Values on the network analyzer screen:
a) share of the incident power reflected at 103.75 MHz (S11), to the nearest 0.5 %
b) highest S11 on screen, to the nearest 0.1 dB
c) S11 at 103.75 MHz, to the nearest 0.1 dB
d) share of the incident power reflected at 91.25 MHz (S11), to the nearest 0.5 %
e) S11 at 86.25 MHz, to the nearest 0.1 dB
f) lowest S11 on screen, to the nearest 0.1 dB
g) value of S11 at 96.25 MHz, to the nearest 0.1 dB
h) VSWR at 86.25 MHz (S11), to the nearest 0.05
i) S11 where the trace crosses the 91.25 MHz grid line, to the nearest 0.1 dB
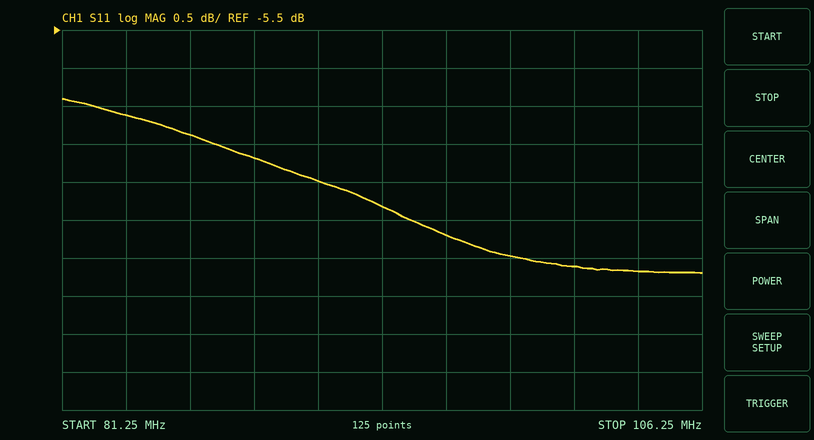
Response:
13.5 %
-6.4 dB
-8.7 dB
18.0 %
-6.9 dB
-8.7 dB
-8.2 dB
2.65
-7.5 dB
